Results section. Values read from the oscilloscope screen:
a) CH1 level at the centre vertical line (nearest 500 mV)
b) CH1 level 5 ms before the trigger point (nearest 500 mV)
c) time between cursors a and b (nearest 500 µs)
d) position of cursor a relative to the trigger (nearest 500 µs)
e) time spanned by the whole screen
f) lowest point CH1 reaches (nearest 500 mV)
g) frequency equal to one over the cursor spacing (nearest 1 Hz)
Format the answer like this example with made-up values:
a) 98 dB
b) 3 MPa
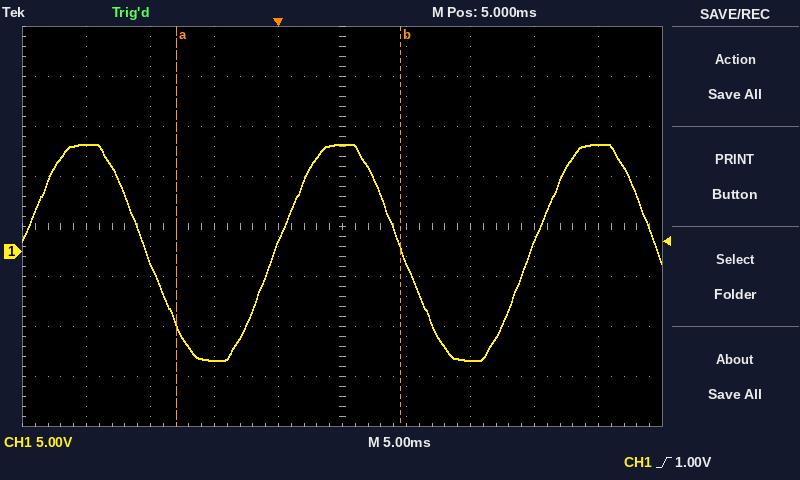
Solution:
a) 10.5 V
b) -11.0 V
c) 17.5 ms
d) -8.0 ms
e) 50 ms
f) -11.0 V
g) 57 Hz
